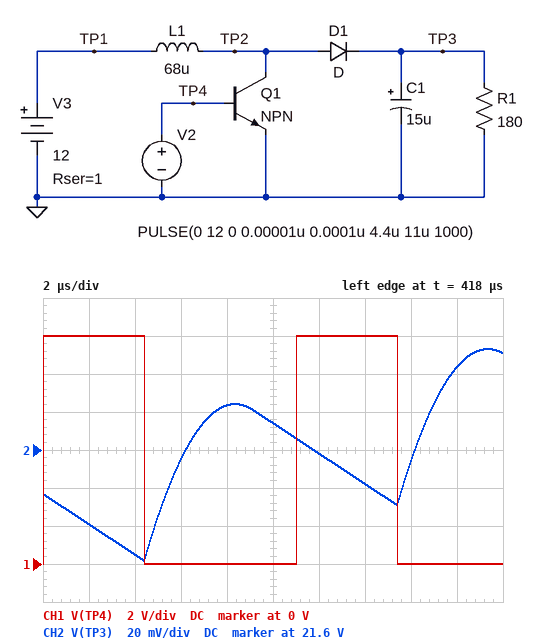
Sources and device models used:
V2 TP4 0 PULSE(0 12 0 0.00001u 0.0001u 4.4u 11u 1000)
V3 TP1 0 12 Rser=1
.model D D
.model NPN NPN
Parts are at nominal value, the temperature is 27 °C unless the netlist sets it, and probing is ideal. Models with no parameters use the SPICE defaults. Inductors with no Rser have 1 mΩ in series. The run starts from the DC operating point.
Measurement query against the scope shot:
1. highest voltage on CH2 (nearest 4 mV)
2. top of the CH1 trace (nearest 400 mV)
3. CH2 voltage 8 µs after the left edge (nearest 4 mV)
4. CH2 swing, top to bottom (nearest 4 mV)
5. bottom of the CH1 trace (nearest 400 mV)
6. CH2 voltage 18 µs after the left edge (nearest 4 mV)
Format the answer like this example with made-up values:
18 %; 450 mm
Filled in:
21.652 V; 12.0 V; 21.624 V; 112 mV; 0 V; 21.644 V
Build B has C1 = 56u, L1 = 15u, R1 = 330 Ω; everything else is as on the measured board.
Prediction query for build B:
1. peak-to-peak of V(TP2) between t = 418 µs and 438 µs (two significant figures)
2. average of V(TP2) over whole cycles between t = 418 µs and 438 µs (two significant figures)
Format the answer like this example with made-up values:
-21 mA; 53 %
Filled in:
20 V; 11 V
